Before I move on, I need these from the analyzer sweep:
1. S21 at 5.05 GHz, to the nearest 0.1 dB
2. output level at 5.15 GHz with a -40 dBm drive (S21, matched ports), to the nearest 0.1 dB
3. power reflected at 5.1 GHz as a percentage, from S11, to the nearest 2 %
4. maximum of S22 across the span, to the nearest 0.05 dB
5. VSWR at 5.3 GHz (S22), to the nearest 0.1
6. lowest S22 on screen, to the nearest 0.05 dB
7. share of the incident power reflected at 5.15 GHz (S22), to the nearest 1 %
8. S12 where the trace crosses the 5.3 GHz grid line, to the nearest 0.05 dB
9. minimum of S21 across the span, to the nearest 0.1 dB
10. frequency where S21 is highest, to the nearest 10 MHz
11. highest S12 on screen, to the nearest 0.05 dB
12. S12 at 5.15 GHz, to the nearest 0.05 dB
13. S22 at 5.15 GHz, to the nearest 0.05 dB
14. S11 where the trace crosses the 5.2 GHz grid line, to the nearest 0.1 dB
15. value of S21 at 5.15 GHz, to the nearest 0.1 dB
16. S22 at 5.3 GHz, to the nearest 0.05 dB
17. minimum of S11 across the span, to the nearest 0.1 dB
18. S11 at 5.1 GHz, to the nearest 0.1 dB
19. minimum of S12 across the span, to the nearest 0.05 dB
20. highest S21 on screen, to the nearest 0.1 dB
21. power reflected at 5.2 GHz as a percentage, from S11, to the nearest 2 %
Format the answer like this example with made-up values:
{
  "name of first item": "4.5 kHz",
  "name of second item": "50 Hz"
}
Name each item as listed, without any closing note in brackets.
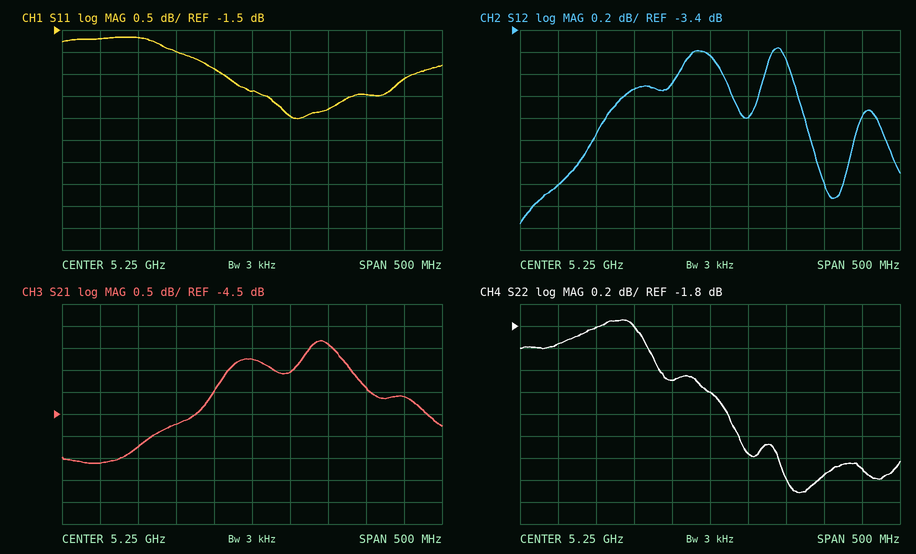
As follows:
{
  "S21 at 5.05 GHz, to the nearest 0.1 dB": "-5.6 dB",
  "output level at 5.15 GHz with a -40 dBm drive (S21, matched ports), to the nearest 0.1 dB": "-44.7 dBm",
  "power reflected at 5.1 GHz as a percentage, from S11, to the nearest 2 %": "68 %",
  "maximum of S22 across the span, to the nearest 0.05 dB": "-1.75 dB",
  "VSWR at 5.3 GHz (S22), to the nearest 0.1": "5.9",
  "lowest S22 on screen, to the nearest 0.05 dB": "-3.30 dB",
  "share of the incident power reflected at 5.15 GHz (S22), to the nearest 1 %": "66 %",
  "S12 where the trace crosses the 5.3 GHz grid line, to the nearest 0.05 dB": "-4.20 dB",
  "minimum of S21 across the span, to the nearest 0.1 dB": "-5.6 dB",
  "frequency where S21 is highest, to the nearest 10 MHz": "5.34 GHz",
  "highest S12 on screen, to the nearest 0.05 dB": "-3.55 dB",
  "S12 at 5.15 GHz, to the nearest 0.05 dB": "-3.95 dB",
  "S22 at 5.15 GHz, to the nearest 0.05 dB": "-1.80 dB",
  "S11 where the trace crosses the 5.2 GHz grid line, to the nearest 0.1 dB": "-2.4 dB",
  "value of S21 at 5.15 GHz, to the nearest 0.1 dB": "-4.7 dB",
  "S22 at 5.3 GHz, to the nearest 0.05 dB": "-2.95 dB",
  "minimum of S11 across the span, to the nearest 0.1 dB": "-3.5 dB",
  "S11 at 5.1 GHz, to the nearest 0.1 dB": "-1.7 dB",
  "minimum of S12 across the span, to the nearest 0.05 dB": "-5.15 dB",
  "highest S21 on screen, to the nearest 0.1 dB": "-2.8 dB",
  "power reflected at 5.2 GHz as a percentage, from S11, to the nearest 2 %": "58 %"
}
